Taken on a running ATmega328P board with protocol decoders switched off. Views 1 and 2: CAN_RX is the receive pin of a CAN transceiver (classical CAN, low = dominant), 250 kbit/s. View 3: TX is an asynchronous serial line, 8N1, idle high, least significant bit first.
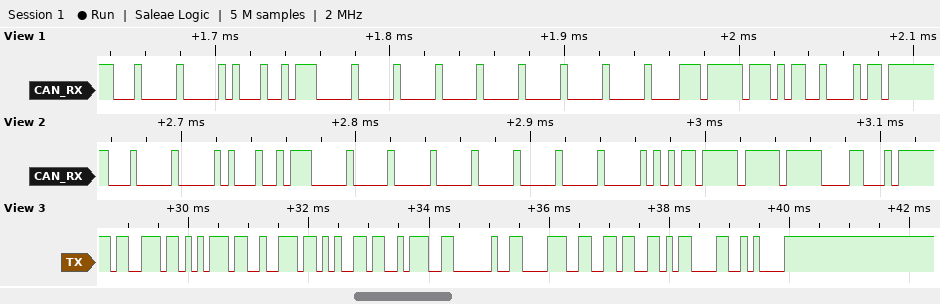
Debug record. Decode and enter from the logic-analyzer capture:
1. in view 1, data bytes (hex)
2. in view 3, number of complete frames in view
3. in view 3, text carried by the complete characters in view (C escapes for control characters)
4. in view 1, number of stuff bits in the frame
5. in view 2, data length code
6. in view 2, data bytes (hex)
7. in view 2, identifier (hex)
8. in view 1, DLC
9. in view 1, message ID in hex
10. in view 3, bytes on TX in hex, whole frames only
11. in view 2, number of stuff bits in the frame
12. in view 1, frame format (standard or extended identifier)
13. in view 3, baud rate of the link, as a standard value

97 00 00 00 00 00 0E FF
10
"sure: 86\r\n"
11
8
97 00 00 00 00 00 56 FF
0x100
8
0x100
73 75 72 65 3A 20 38 36 0D 0A
13
standard
9600 baud
